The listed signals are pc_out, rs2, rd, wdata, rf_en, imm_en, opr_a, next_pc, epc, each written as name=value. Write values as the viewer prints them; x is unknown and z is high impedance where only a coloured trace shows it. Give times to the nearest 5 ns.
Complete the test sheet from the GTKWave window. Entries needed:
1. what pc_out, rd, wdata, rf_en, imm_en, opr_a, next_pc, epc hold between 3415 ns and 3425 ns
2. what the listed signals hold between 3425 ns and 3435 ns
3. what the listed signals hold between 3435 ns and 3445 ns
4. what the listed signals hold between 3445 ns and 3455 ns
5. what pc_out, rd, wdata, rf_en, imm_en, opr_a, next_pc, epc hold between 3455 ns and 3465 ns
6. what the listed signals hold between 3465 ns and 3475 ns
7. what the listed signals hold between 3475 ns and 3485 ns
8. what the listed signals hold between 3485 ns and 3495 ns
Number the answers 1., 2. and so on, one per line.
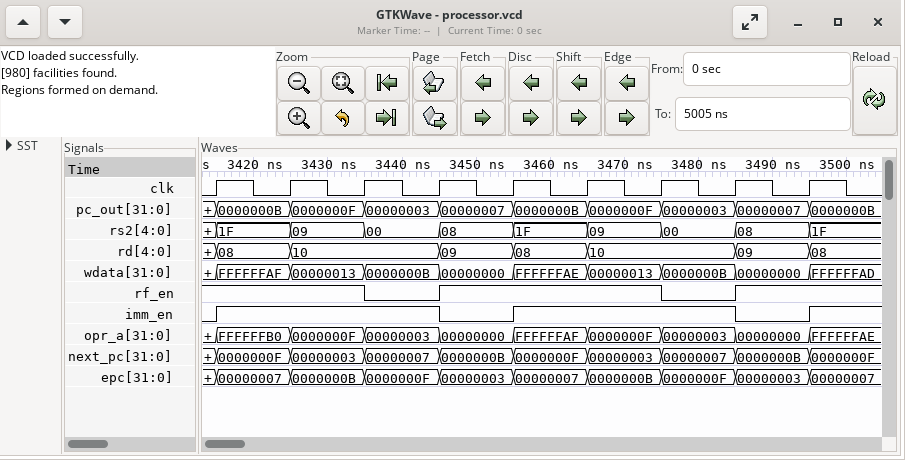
1. pc_out=0000000B, rd=08, wdata=FFFFFFAF, rf_en=1, imm_en=1, opr_a=FFFFFFB0, next_pc=0000000F, epc=00000007
2. pc_out=0000000F, rs2=09, rd=10, wdata=00000013, rf_en=1, imm_en=1, opr_a=0000000F, next_pc=00000003, epc=0000000B
3. pc_out=00000003, rs2=00, rd=10, wdata=0000000B, rf_en=0, imm_en=1, opr_a=00000003, next_pc=00000007, epc=0000000F
4. pc_out=00000007, rs2=08, rd=09, wdata=00000000, rf_en=1, imm_en=0, opr_a=00000000, next_pc=0000000B, epc=00000003
5. pc_out=0000000B, rd=08, wdata=FFFFFFAE, rf_en=1, imm_en=1, opr_a=FFFFFFAF, next_pc=0000000F, epc=00000007
6. pc_out=0000000F, rs2=09, rd=10, wdata=00000013, rf_en=1, imm_en=1, opr_a=0000000F, next_pc=00000003, epc=0000000B
7. pc_out=00000003, rs2=00, rd=10, wdata=0000000B, rf_en=0, imm_en=1, opr_a=00000003, next_pc=00000007, epc=0000000F
8. pc_out=00000007, rs2=08, rd=09, wdata=00000000, rf_en=1, imm_en=0, opr_a=00000000, next_pc=0000000B, epc=00000003
